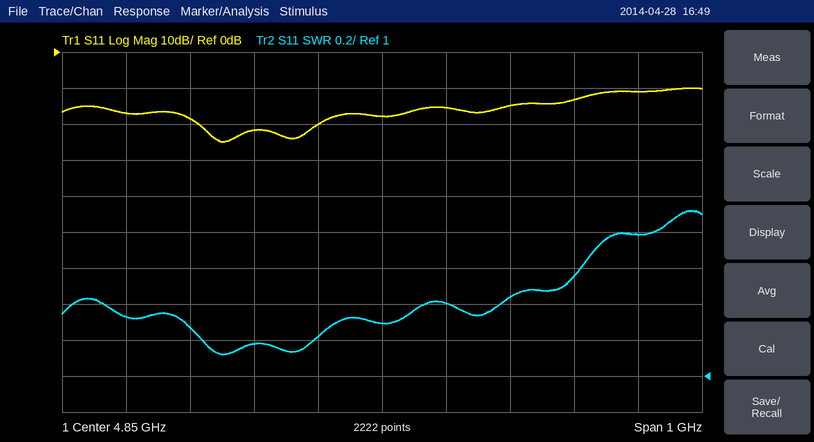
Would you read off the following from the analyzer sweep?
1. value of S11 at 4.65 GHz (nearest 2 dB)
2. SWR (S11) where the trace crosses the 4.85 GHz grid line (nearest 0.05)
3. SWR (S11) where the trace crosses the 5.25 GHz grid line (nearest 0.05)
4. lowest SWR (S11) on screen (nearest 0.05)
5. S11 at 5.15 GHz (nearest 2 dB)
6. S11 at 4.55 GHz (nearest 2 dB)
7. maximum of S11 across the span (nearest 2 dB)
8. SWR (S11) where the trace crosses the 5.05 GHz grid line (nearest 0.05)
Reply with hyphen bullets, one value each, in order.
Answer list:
- -22 dB
- 1.30
- 1.80
- 1.10
- -14 dB
- -18 dB
- -10 dB
- 1.45
